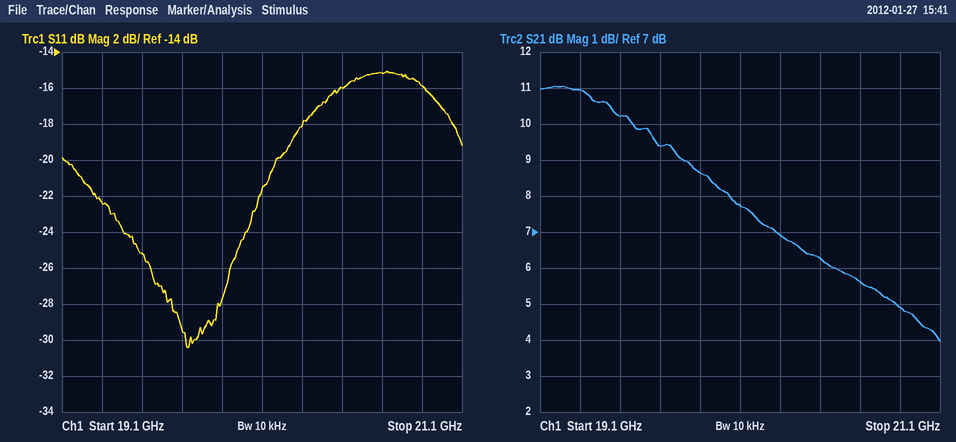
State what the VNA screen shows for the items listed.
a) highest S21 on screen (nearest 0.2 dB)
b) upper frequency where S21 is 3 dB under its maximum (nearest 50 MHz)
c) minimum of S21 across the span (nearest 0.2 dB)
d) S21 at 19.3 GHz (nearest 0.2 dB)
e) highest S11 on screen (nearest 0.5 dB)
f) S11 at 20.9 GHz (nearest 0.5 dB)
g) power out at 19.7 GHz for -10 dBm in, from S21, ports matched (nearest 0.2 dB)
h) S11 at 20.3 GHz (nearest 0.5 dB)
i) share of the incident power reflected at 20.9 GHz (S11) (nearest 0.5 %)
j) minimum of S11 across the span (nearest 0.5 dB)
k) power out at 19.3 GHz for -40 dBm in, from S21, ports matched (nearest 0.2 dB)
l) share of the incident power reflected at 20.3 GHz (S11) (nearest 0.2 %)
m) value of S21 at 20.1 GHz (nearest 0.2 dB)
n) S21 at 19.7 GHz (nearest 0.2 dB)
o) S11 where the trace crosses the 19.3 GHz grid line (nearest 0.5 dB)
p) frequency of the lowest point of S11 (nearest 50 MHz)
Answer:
11.0 dB
20.05 GHz
4.0 dB
11.0 dB
-15.0 dB
-16.0 dB
-0.6 dBm
-18.0 dB
2.5 %
-30.5 dB
-29.0 dBm
1.6 %
7.8 dB
9.4 dB
-22.5 dB
19.75 GHz
